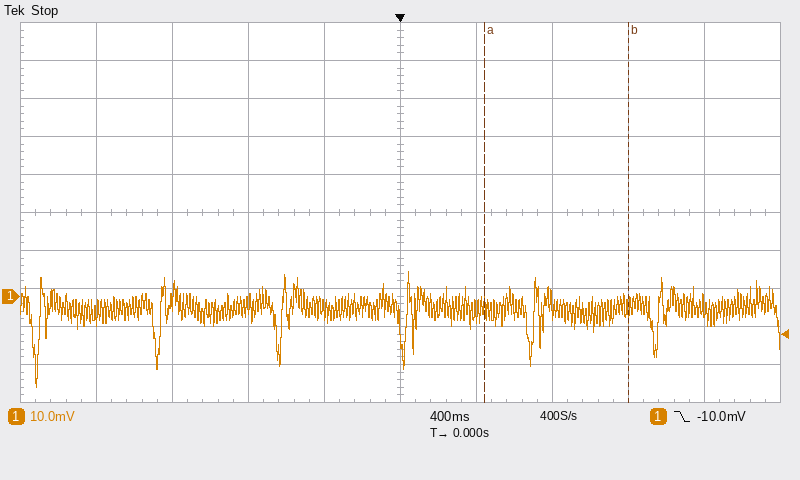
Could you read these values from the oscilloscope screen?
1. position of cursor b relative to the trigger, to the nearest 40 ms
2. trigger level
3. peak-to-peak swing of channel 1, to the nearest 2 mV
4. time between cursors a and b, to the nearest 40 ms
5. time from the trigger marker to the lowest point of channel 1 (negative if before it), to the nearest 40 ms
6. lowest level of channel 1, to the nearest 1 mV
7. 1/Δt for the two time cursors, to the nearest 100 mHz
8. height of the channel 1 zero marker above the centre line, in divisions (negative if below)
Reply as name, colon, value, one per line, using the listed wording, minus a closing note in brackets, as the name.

position of cursor b relative to the trigger, to the nearest 40 ms: +1.20 s
trigger level: -10.0 mV
peak-to-peak swing of channel 1, to the nearest 2 mV: 30 mV
time between cursors a and b, to the nearest 40 ms: 760 ms
time from the trigger marker to the lowest point of channel 1 (negative if before it), to the nearest 40 ms: -1.92 s
lowest level of channel 1, to the nearest 1 mV: -24 mV
1/Δt for the two time cursors, to the nearest 100 mHz: 1.3 Hz
height of the channel 1 zero marker above the centre line, in divisions: -2.2 div
